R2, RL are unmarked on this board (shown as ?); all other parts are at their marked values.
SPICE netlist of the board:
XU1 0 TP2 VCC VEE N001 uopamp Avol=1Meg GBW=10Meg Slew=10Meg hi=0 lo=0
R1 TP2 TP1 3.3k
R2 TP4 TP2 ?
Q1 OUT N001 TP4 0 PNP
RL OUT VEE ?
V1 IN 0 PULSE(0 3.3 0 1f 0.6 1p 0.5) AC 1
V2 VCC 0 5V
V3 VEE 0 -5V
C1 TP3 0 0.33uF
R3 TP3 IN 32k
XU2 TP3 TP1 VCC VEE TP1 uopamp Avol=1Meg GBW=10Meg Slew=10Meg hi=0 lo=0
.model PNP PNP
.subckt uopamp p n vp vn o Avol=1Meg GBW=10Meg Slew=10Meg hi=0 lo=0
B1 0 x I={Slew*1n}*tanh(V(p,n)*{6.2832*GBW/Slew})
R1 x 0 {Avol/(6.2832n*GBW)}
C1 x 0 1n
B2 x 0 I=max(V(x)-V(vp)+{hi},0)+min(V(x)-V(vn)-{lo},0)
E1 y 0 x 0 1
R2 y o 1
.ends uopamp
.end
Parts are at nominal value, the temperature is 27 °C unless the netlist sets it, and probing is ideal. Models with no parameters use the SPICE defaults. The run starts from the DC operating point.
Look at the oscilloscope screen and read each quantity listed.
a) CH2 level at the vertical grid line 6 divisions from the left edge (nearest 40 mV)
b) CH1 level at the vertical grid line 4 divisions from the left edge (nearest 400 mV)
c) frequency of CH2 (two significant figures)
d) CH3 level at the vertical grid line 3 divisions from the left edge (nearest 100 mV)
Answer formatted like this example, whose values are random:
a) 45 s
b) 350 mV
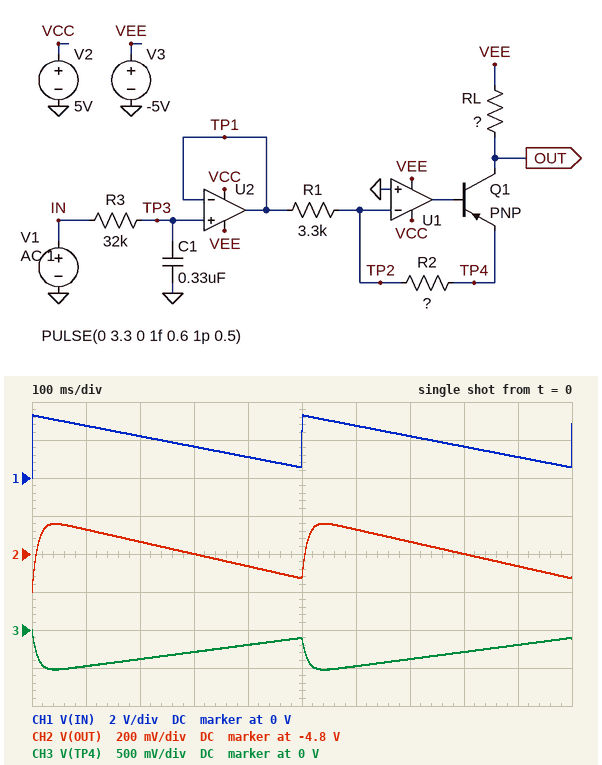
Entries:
a) -4.68 V
b) 1.2 V
c) 2.0 Hz
d) -300 mV
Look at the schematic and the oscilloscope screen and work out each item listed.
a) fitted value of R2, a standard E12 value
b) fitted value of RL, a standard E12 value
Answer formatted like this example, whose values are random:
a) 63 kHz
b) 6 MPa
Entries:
a) 560 Ω
b) 390 Ω
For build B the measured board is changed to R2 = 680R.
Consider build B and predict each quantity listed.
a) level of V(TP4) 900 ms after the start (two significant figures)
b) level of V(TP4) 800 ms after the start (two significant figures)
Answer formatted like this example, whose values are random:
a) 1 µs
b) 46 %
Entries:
a) -240 mV
b) -350 mV
